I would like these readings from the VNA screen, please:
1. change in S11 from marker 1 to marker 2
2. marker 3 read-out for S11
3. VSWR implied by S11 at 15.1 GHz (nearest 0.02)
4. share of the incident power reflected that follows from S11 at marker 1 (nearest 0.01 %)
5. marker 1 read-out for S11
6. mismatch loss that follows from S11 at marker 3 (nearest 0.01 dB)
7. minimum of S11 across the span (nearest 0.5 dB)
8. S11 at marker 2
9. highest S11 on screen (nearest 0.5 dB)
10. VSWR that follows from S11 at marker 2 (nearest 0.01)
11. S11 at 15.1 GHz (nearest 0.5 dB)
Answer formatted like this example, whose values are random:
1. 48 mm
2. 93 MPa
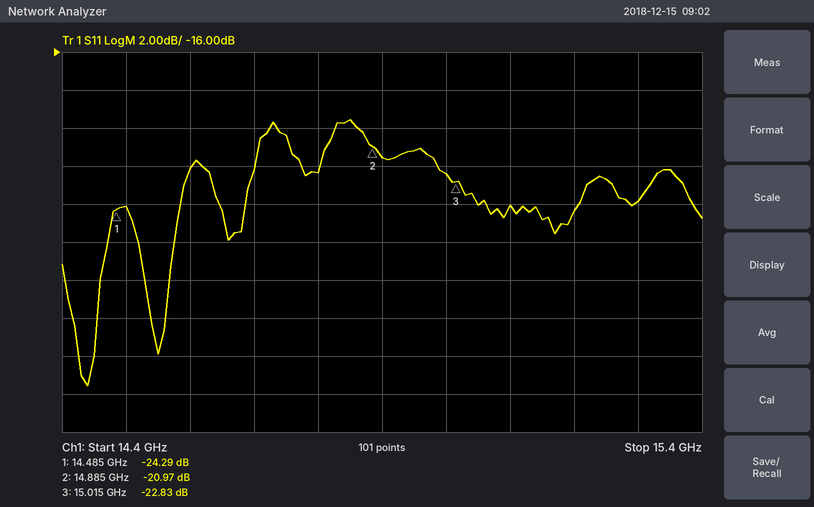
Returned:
1. 3.32 dB
2. -22.83 dB
3. 1.14
4. 0.37 %
5. -24.29 dB
6. 0.02 dB
7. -33.5 dB
8. -20.97 dB
9. -19.5 dB
10. 1.20
11. -24.0 dB
